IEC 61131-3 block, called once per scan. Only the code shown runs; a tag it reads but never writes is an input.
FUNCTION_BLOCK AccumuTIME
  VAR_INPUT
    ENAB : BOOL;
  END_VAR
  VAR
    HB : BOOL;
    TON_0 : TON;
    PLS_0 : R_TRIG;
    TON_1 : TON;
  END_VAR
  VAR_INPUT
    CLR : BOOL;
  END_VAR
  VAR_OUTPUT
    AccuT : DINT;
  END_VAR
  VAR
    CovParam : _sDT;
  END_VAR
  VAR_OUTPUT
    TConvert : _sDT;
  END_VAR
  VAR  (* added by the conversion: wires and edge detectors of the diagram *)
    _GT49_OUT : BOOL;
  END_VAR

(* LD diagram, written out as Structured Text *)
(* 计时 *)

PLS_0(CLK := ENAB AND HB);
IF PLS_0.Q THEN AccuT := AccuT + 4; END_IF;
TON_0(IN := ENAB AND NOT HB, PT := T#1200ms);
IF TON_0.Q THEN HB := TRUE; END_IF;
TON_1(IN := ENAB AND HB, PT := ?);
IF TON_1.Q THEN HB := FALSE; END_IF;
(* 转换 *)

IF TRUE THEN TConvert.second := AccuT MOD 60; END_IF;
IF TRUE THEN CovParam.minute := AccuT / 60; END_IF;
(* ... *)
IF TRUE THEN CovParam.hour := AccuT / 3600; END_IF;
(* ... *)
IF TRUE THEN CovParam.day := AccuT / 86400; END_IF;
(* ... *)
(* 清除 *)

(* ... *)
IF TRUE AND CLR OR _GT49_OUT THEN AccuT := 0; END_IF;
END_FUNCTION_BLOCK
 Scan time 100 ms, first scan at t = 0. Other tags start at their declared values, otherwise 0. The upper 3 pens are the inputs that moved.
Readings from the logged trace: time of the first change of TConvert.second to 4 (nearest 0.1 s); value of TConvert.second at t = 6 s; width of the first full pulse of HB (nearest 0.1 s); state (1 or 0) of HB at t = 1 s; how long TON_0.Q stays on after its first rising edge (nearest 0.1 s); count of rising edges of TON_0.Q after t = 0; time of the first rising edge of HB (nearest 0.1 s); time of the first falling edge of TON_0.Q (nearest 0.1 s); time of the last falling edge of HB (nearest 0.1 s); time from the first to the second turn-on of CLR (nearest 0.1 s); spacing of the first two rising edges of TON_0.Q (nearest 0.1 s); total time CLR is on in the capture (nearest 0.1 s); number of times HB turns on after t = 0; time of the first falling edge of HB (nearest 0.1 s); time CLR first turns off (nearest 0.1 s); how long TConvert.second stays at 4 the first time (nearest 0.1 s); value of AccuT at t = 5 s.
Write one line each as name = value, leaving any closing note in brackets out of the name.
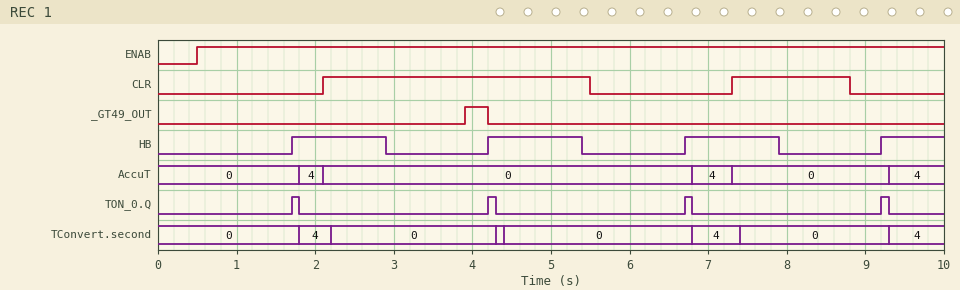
time of the first change of TConvert.second to 4 = 1.8 s
value of TConvert.second at t = 6 s = 0
width of the first full pulse of HB = 1.2 s
state (1 or 0) of HB at t = 1 s = 0
how long TON_0.Q stays on after its first rising edge = 0.1 s
count of rising edges of TON_0.Q after t = 0 = 4
time of the first rising edge of HB = 1.7 s
time of the first falling edge of TON_0.Q = 1.8 s
time of the last falling edge of HB = 7.9 s
time from the first to the second turn-on of CLR = 5.2 s
spacing of the first two rising edges of TON_0.Q = 2.5 s
total time CLR is on in the capture = 4.9 s
number of times HB turns on after t = 0 = 4
time of the first falling edge of HB = 2.9 s
time CLR first turns off = 5.5 s
how long TConvert.second stays at 4 the first time = 0.4 s
value of AccuT at t = 5 s = 0
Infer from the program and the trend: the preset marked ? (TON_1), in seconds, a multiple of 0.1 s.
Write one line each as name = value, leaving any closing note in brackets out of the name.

the preset marked ? (TON_1), in seconds, a multiple of 0.1 s = 1.2 s
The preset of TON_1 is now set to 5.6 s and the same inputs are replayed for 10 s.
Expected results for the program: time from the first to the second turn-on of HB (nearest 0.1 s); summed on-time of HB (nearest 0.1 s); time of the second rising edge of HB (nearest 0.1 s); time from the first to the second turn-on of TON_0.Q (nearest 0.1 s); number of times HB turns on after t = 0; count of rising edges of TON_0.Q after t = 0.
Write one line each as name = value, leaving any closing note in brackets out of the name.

time from the first to the second turn-on of HB = 6.9 s
summed on-time of HB = 7.0 s
time of the second rising edge of HB = 8.6 s
time from the first to the second turn-on of TON_0.Q = 6.9 s
number of times HB turns on after t = 0 = 2
count of rising edges of TON_0.Q after t = 0 = 2
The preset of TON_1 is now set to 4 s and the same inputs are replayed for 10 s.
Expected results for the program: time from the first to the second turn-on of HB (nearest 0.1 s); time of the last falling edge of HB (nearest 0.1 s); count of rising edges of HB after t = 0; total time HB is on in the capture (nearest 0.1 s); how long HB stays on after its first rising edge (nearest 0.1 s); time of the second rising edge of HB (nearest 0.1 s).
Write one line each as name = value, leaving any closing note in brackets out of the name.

time from the first to the second turn-on of HB = 5.3 s
time of the last falling edge of HB = 5.7 s
count of rising edges of HB after t = 0 = 2
total time HB is on in the capture = 7.0 s
how long HB stays on after its first rising edge = 4.0 s
time of the second rising edge of HB = 7.0 s
